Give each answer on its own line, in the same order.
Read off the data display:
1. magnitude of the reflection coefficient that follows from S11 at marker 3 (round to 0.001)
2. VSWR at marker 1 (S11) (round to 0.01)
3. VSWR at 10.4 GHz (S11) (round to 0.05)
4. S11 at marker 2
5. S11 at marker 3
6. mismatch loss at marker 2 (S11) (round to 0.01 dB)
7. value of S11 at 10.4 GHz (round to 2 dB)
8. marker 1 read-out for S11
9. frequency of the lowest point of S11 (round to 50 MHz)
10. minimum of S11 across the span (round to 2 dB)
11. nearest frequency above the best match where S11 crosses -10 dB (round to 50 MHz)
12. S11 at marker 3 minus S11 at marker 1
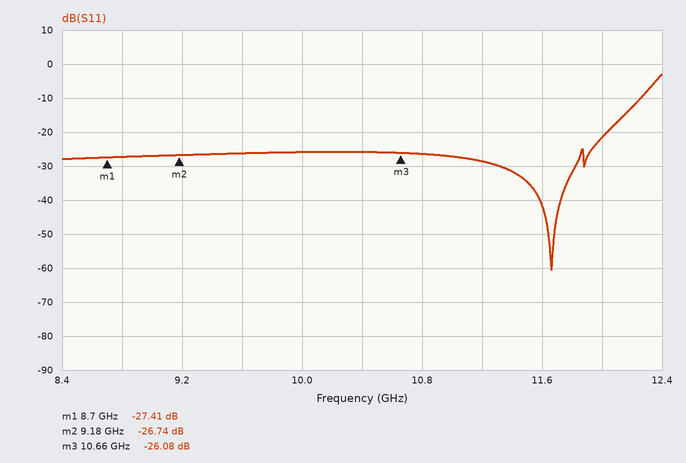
0.050
1.09
1.10
-26.74 dB
-26.08 dB
0.01 dB
-26 dB
-27.41 dB
11.65 GHz
-60 dB
12.25 GHz
1.33 dB
